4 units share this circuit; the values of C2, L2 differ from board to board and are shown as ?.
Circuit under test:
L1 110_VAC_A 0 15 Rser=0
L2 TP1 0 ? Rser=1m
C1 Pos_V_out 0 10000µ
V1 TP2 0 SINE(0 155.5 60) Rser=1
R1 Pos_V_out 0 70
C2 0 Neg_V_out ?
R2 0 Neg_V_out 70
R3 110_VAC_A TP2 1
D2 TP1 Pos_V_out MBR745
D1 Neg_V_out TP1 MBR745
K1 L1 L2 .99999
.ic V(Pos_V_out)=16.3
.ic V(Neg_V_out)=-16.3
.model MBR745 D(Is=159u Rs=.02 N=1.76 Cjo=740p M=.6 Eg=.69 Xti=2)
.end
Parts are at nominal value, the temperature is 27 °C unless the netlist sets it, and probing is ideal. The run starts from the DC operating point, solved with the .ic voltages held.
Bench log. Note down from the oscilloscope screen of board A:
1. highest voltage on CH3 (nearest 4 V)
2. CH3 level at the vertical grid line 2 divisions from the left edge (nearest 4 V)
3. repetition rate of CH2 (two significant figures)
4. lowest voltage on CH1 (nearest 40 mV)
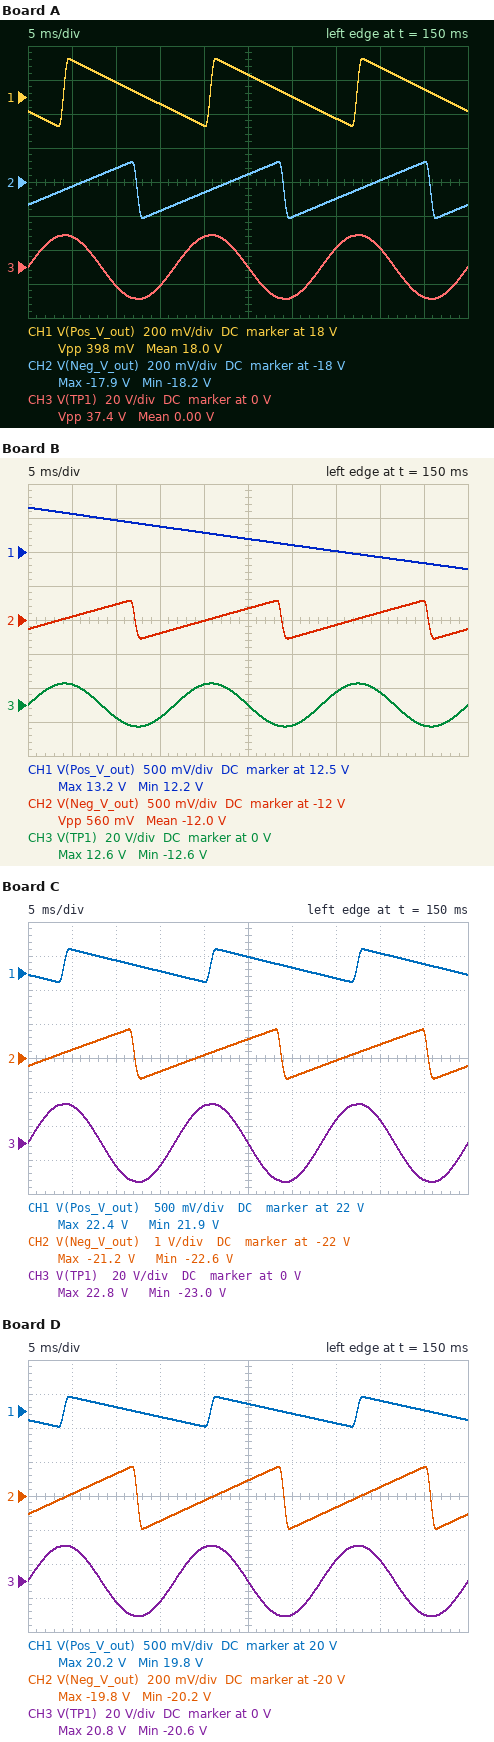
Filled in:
20 V
-12 V
60 Hz
17.84 V
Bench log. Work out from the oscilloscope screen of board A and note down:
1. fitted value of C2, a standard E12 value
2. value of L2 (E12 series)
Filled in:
12 mF
220 mH
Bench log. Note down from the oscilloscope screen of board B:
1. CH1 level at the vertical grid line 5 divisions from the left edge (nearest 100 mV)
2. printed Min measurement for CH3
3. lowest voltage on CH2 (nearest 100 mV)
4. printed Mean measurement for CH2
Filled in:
12.7 V
-12.6 V
-12.3 V
-12.0 V
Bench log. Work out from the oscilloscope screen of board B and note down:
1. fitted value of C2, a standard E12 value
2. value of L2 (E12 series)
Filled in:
4.7 mF
100 mH
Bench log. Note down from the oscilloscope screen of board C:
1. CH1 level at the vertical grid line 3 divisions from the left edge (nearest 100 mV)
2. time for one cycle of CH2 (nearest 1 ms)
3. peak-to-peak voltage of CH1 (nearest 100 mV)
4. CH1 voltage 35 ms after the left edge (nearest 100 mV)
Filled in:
22.0 V
17 ms
500 mV
21.9 V
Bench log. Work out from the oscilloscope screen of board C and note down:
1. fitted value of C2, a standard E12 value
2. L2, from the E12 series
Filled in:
3.3 mF
330 mH
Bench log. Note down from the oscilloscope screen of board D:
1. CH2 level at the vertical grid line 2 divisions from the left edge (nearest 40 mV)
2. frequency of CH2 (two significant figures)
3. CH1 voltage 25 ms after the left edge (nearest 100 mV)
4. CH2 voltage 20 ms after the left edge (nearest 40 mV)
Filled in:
-19.88 V
60 Hz
20.1 V
-20.04 V
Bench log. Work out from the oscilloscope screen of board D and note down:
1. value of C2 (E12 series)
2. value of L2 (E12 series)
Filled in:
12 mF
270 mH
